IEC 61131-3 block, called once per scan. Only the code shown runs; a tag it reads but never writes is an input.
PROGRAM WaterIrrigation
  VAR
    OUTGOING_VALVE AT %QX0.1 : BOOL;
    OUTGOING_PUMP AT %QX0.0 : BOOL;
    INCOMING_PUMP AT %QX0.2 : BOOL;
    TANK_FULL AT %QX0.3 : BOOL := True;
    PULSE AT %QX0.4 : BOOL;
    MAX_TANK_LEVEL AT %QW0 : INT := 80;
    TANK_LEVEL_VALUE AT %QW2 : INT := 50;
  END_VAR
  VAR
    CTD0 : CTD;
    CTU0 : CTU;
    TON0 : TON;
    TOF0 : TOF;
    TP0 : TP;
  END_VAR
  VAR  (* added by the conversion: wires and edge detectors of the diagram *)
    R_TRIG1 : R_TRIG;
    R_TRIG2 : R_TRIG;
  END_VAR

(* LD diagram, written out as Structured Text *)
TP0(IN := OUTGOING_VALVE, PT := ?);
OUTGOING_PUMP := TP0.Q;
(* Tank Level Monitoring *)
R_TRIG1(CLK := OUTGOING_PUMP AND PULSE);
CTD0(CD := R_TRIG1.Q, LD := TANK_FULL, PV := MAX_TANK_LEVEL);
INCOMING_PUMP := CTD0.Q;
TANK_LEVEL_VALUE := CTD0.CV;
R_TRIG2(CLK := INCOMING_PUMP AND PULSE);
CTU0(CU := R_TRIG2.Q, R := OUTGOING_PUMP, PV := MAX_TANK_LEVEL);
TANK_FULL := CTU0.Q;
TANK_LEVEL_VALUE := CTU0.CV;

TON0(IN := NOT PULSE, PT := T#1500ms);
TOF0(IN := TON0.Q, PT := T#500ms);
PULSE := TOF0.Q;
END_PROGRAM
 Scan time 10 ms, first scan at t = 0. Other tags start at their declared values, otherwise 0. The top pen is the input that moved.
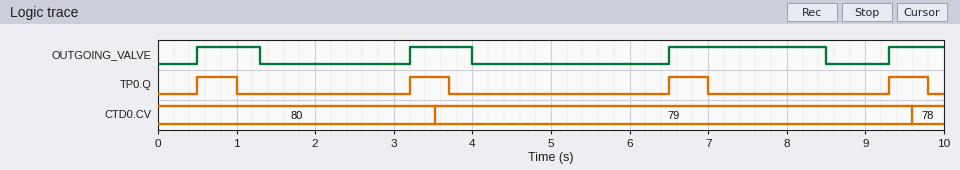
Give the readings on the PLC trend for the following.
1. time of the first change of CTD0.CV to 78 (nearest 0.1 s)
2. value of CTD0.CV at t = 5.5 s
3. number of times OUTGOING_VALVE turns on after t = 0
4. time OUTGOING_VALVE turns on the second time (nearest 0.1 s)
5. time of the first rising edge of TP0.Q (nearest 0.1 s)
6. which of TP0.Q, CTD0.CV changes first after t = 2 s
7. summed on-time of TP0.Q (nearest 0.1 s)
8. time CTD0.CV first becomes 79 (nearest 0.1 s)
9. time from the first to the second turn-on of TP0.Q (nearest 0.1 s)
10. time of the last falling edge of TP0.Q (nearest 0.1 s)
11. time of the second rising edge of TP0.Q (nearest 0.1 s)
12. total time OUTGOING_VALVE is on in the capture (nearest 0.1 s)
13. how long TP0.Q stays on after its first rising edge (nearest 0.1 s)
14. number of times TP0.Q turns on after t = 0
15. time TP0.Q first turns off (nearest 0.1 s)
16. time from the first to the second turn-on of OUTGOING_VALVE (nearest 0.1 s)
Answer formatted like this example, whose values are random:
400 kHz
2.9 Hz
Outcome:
9.6 s
79
4
3.2 s
0.5 s
TP0.Q
2.0 s
3.5 s
2.7 s
9.8 s
3.2 s
4.3 s
0.5 s
4
1.0 s
2.7 s
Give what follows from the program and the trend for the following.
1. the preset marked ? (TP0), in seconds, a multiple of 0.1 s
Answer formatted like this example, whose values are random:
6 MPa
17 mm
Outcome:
0.5 s
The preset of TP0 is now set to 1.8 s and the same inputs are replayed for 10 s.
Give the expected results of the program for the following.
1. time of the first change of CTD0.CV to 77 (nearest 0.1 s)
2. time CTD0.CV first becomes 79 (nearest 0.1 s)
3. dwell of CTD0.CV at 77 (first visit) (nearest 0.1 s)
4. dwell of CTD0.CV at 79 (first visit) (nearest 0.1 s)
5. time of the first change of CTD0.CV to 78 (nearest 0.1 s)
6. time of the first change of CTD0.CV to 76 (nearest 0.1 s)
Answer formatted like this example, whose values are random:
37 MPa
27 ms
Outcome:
7.6 s
1.5 s
2.0 s
2.0 s
3.5 s
9.6 s
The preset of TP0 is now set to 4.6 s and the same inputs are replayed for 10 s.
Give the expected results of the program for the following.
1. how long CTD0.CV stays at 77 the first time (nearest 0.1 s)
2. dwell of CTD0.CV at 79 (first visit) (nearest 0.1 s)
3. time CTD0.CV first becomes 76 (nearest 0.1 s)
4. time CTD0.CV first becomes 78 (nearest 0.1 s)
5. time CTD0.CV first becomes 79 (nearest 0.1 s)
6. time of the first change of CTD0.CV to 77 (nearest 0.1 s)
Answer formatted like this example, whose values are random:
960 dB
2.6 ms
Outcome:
2.0 s
2.0 s
9.6 s
3.5 s
1.5 s
7.6 s
